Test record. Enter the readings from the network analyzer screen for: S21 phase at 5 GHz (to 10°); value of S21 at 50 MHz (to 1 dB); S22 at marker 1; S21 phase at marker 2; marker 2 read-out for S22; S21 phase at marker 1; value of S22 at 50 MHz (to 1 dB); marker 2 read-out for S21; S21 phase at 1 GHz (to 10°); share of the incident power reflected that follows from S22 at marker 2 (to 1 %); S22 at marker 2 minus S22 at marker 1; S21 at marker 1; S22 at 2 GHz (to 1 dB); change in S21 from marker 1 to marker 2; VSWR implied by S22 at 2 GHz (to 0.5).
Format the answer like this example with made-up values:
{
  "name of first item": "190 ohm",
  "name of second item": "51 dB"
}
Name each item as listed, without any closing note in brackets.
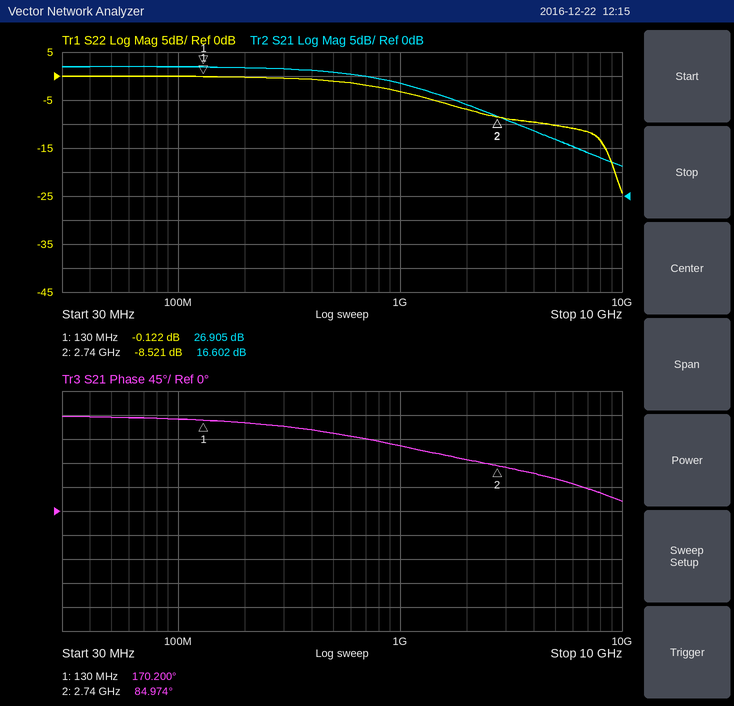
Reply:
{
  "S21 phase at 5 GHz": "60°",
  "value of S21 at 50 MHz": "27 dB",
  "S22 at marker 1": "-0.122 dB",
  "S21 phase at marker 2": "84.974°",
  "marker 2 read-out for S22": "-8.521 dB",
  "S21 phase at marker 1": "170.200°",
  "value of S22 at 50 MHz": "0 dB",
  "marker 2 read-out for S21": "16.602 dB",
  "S21 phase at 1 GHz": "120°",
  "share of the incident power reflected that follows from S22 at marker 2": "14 %",
  "S22 at marker 2 minus S22 at marker 1": "-8.399 dB",
  "S21 at marker 1": "26.905 dB",
  "S22 at 2 GHz": "-7 dB",
  "change in S21 from marker 1 to marker 2": "-10.303 dB",
  "VSWR implied by S22 at 2 GHz": "2.5"
}
